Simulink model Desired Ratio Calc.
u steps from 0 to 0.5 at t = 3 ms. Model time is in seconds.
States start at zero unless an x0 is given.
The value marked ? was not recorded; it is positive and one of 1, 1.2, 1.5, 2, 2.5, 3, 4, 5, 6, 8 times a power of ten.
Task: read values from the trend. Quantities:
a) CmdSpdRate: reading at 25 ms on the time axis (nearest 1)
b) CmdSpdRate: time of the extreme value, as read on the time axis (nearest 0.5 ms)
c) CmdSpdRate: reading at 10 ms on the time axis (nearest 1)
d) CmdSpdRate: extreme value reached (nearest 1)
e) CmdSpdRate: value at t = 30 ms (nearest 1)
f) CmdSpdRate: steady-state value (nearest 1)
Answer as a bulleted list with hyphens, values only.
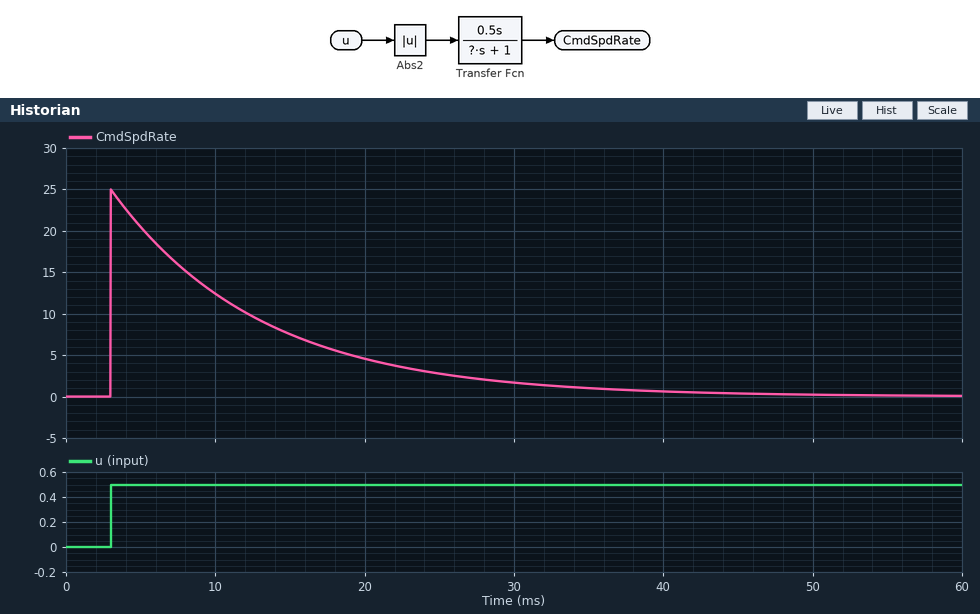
- 3
- 3.0 ms
- 12
- 25
- 2
- 0
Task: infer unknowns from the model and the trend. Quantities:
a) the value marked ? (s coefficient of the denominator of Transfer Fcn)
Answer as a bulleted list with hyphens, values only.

- 0.01
